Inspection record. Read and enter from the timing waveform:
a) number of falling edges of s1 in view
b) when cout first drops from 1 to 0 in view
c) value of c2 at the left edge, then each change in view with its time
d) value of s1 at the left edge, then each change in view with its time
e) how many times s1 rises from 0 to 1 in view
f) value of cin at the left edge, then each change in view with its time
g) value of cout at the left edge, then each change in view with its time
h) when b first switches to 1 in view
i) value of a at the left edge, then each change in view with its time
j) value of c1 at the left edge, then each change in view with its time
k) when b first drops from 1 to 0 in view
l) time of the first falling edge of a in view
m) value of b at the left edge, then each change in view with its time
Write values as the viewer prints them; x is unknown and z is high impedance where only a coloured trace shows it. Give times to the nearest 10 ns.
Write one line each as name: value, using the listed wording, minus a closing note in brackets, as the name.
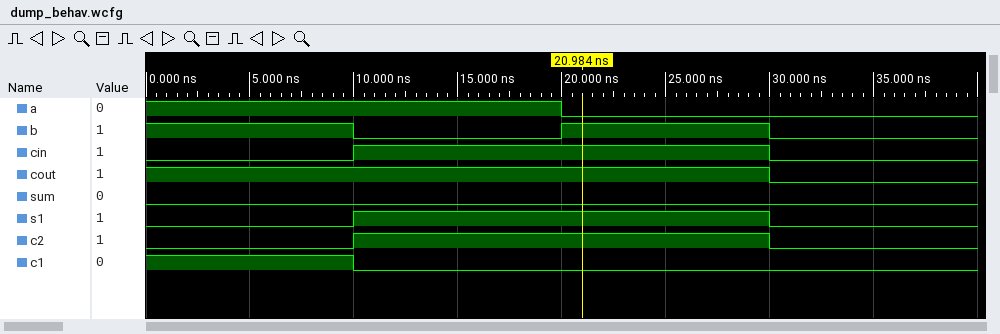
number of falling edges of s1 in view: 1
when cout first drops from 1 to 0 in view: 30 ns
value of c2 at the left edge, then each change in view with its time: 0, 1 at 10 ns, 0 at 30 ns
value of s1 at the left edge, then each change in view with its time: 0, 1 at 10 ns, 0 at 30 ns
how many times s1 rises from 0 to 1 in view: 1
value of cin at the left edge, then each change in view with its time: 0, 1 at 10 ns, 0 at 30 ns
value of cout at the left edge, then each change in view with its time: 1, 0 at 30 ns
when b first switches to 1 in view: 20 ns
value of a at the left edge, then each change in view with its time: 1, 0 at 20 ns
value of c1 at the left edge, then each change in view with its time: 1, 0 at 10 ns
when b first drops from 1 to 0 in view: 10 ns
time of the first falling edge of a in view: 20 ns
value of b at the left edge, then each change in view with its time: 1, 0 at 10 ns, 1 at 20 ns, 0 at 30 ns
